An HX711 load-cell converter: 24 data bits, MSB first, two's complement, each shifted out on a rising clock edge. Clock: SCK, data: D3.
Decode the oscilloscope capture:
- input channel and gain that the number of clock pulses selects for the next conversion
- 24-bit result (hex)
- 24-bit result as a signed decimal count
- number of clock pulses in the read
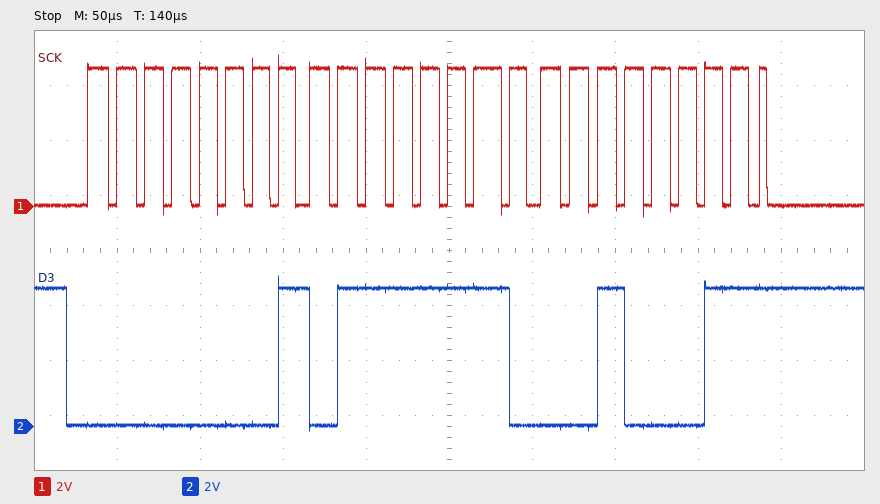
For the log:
channel A, gain 128
0x017E23
97827
25
